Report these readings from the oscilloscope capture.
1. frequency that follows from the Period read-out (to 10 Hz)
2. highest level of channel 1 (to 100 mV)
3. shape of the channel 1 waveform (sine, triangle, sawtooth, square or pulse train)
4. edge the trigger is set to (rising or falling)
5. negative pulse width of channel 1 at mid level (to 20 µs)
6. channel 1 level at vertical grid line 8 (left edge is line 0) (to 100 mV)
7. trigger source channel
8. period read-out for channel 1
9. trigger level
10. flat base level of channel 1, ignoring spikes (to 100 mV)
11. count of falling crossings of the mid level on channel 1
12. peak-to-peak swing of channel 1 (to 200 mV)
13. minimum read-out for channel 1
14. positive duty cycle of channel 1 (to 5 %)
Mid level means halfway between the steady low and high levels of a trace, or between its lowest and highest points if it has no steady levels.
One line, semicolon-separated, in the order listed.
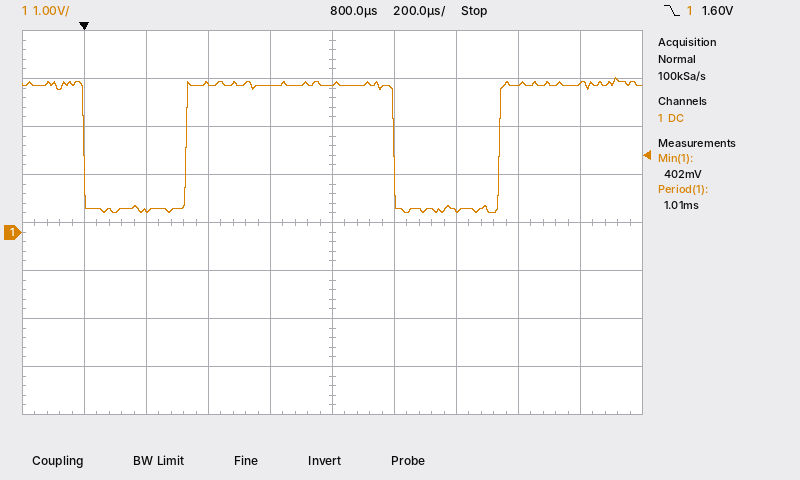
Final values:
990 Hz; 3.2 V; pulse train; falling; 340 µs; 3.1 V; channel 1; 1.01 ms; 1.60 V; 500 mV; 2; 2.8 V; 402 mV; 65 %
